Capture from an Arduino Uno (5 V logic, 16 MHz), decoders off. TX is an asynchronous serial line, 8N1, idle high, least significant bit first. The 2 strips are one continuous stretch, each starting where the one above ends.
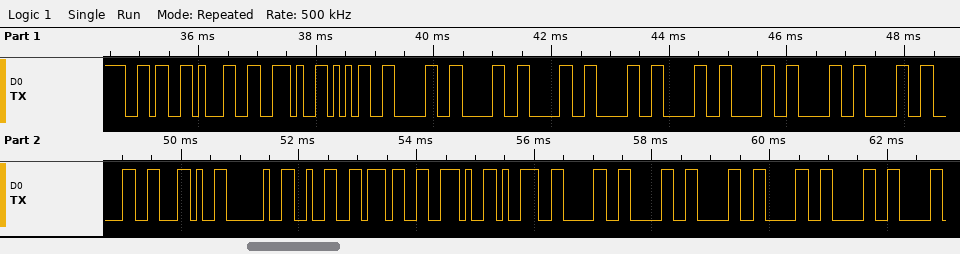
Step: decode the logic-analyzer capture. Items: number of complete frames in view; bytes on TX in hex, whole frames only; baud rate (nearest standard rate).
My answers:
24
36 31 2E 35 30 30 30 30 30 30 30 30 30 2C 20 32 37 2E 39 30 30 30 30 30
9600 baud
